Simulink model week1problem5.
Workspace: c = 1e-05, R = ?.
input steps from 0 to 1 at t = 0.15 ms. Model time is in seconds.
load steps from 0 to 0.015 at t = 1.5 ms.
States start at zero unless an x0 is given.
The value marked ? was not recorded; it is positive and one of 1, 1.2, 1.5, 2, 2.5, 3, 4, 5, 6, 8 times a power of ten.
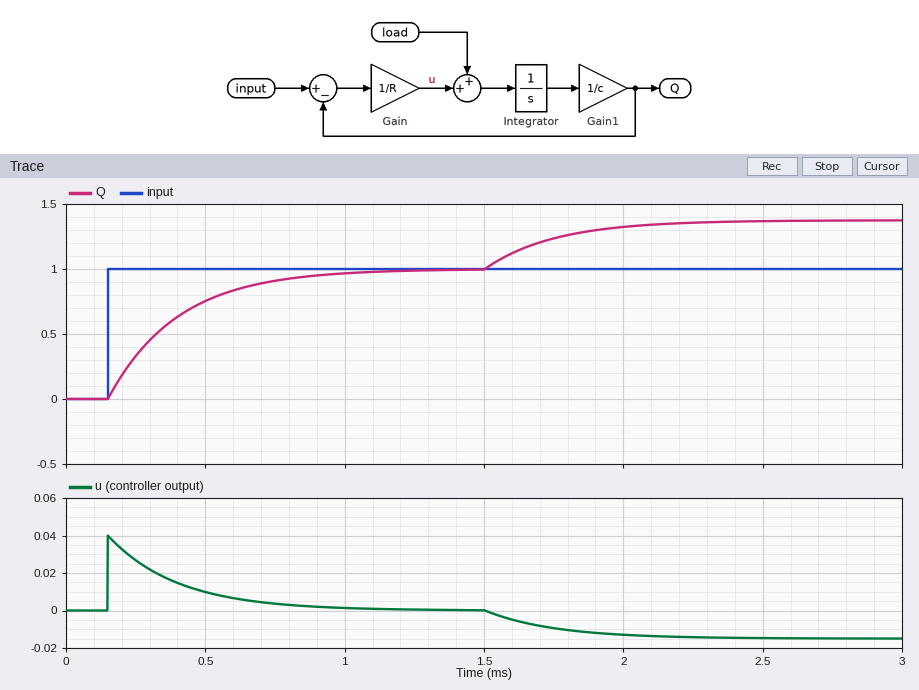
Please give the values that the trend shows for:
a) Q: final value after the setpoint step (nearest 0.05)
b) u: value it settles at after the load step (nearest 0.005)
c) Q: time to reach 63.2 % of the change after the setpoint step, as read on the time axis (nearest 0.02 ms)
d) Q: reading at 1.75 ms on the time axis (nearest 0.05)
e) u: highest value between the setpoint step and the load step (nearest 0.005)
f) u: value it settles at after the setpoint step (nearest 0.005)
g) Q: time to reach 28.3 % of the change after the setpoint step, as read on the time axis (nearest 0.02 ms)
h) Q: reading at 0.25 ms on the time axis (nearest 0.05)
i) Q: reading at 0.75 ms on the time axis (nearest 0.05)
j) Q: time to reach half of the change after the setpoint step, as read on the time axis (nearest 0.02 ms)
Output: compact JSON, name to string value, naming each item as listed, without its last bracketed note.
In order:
{"Q: final value after the setpoint step": "1.00", "u: value it settles at after the load step": "-0.015", "Q: time to reach 63.2 % of the change after the setpoint step, as read on the time axis": "0.40 ms", "Q: reading at 1.75 ms on the time axis": "1.25", "u: highest value between the setpoint step and the load step": "0.040", "u: value it settles at after the setpoint step": "0.000", "Q: time to reach 28.3 % of the change after the setpoint step, as read on the time axis": "0.24 ms", "Q: reading at 0.25 ms on the time axis": "0.35", "Q: reading at 0.75 ms on the time axis": "0.90", "Q: time to reach half of the change after the setpoint step, as read on the time axis": "0.32 ms"}
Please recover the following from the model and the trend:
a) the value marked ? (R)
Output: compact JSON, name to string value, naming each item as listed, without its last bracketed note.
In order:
{"the value marked ?": "25"}
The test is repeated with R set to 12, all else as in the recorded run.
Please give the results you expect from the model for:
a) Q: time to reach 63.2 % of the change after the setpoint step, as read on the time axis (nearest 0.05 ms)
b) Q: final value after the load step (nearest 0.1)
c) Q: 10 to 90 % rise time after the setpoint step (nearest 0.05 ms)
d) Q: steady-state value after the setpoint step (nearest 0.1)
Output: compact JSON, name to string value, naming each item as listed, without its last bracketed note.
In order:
{"Q: time to reach 63.2 % of the change after the setpoint step, as read on the time axis": "0.25 ms", "Q: final value after the load step": "1.2", "Q: 10 to 90 % rise time after the setpoint step": "0.25 ms", "Q: steady-state value after the setpoint step": "1.0"}
